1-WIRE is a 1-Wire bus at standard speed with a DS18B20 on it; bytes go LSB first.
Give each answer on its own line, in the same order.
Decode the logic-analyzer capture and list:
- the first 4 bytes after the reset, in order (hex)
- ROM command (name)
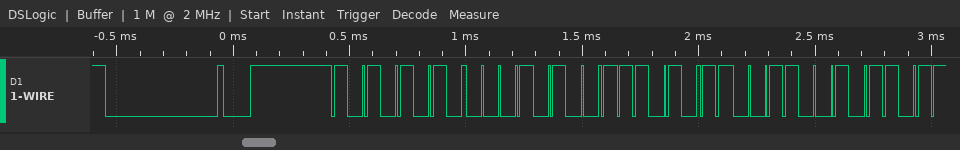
55 28 D7 4C
Match ROM
